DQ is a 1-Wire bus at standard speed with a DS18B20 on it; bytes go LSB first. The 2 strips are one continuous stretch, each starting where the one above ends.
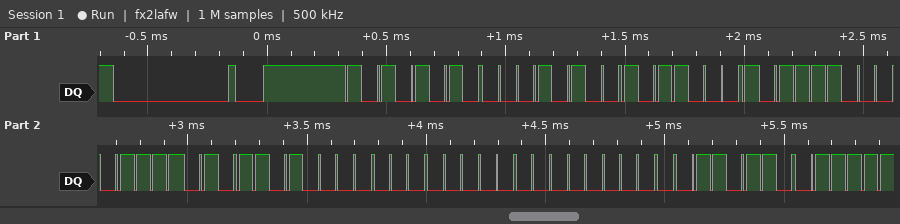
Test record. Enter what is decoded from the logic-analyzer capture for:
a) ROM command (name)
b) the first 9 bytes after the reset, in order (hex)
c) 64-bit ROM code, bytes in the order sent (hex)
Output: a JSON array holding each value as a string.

["Match ROM", "55 28 8D 1E 5E 0B 00 00 6C", "28 8D 1E 5E 0B 00 00 6C"]
